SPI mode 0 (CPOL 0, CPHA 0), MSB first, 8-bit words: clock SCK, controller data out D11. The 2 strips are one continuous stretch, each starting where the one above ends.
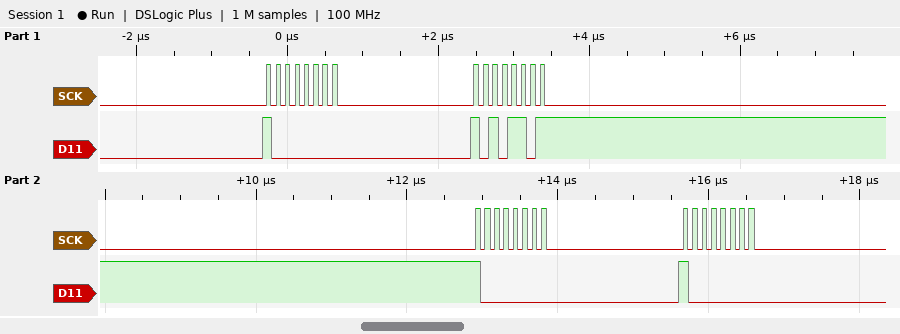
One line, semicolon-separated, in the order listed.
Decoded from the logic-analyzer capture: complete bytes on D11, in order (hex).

80 AD 80 80
